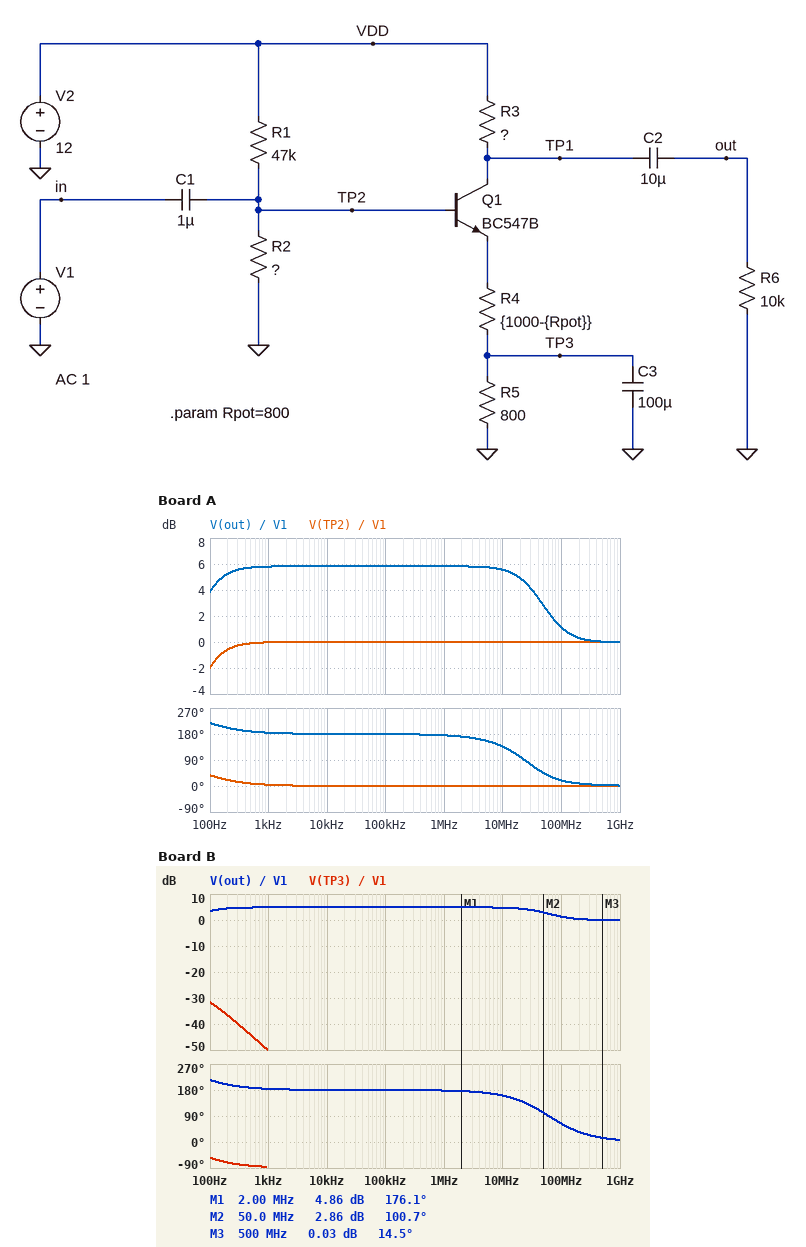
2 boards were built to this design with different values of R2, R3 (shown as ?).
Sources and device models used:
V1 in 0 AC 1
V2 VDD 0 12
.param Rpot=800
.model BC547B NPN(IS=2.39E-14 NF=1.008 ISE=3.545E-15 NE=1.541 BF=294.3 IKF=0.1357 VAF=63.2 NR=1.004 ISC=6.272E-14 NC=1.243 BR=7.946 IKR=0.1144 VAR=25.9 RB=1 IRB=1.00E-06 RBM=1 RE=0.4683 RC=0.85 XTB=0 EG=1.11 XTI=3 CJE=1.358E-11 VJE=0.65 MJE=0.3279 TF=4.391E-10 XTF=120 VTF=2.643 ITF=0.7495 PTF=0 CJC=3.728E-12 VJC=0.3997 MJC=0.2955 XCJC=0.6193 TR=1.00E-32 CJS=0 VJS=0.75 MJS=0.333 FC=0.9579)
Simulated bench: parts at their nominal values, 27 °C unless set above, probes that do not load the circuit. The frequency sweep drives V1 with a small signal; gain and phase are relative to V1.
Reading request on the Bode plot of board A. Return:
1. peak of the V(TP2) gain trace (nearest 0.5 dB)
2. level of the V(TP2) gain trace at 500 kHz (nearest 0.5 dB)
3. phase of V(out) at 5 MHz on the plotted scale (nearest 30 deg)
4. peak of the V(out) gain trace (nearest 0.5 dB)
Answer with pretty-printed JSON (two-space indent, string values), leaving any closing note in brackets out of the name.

{
  "peak of the V(TP2) gain trace": "0 dB",
  "level of the V(TP2) gain trace at 500 kHz": "0 dB",
  "phase of V(out) at 5 MHz on the plotted scale": "150 deg",
  "peak of the V(out) gain trace": "6.0 dB"
}
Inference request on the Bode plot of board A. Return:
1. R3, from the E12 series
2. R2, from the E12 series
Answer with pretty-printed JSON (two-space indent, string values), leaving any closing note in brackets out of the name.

{
  "R3, from the E12 series": "6.8 kΩ",
  "R2, from the E12 series": "2.2 kΩ"
}
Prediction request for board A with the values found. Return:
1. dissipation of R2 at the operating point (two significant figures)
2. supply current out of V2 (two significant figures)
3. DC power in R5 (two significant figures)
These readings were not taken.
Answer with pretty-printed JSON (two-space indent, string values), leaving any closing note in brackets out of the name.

{
  "dissipation of R2 at the operating point": "130 µW",
  "supply current out of V2": "260 µA",
  "DC power in R5": "160 nW"
}
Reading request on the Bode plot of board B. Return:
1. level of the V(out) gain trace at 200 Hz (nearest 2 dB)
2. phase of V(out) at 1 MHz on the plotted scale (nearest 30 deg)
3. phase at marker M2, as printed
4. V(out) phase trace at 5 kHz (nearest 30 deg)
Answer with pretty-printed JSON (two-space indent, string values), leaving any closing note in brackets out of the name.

{
  "level of the V(out) gain trace at 200 Hz": "4 dB",
  "phase of V(out) at 1 MHz on the plotted scale": "180 deg",
  "phase at marker M2, as printed": "100.7 deg",
  "V(out) phase trace at 5 kHz": "180 deg"
}
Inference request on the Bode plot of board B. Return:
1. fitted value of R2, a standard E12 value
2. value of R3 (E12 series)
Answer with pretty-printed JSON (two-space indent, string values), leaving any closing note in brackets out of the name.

{
  "fitted value of R2, a standard E12 value": "2.7 kΩ",
  "value of R3": "1 kΩ"
}
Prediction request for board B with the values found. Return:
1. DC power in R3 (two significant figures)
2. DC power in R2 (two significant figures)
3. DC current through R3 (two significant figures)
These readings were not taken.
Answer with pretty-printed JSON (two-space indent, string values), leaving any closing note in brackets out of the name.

{
  "DC power in R3": "6.8 µW",
  "DC power in R2": "160 µW",
  "DC current through R3": "82 µA"
}
